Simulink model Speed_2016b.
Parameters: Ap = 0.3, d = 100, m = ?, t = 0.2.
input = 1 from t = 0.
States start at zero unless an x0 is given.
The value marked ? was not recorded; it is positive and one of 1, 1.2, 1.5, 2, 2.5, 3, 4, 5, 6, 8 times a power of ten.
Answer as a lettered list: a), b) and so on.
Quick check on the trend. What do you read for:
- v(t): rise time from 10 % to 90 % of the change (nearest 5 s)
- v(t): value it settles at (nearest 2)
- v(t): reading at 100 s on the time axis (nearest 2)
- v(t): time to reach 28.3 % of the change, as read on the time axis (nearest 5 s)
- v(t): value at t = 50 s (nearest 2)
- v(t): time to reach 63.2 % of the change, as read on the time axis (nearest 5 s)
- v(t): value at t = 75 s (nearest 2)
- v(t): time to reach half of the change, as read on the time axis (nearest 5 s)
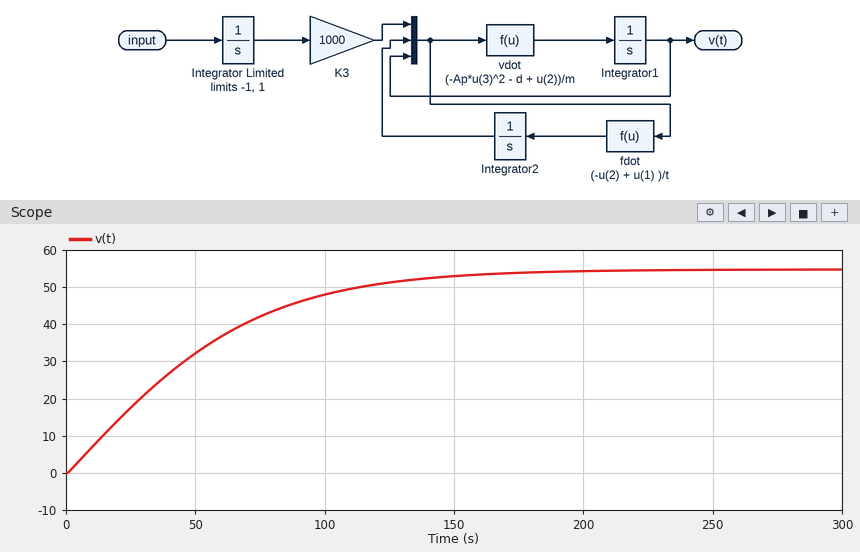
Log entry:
a) 100 s
b) 54
c) 48
d) 20 s
e) 32
f) 55 s
g) 42
h) 40 s
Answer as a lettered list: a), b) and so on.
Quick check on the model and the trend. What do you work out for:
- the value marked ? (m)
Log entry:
a) 1200
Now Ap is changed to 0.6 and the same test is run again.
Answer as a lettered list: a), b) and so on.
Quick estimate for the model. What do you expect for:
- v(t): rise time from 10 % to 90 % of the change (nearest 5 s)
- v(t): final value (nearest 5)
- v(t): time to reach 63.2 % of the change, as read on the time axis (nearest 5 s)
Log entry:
a) 70 s
b) 40
c) 40 s
